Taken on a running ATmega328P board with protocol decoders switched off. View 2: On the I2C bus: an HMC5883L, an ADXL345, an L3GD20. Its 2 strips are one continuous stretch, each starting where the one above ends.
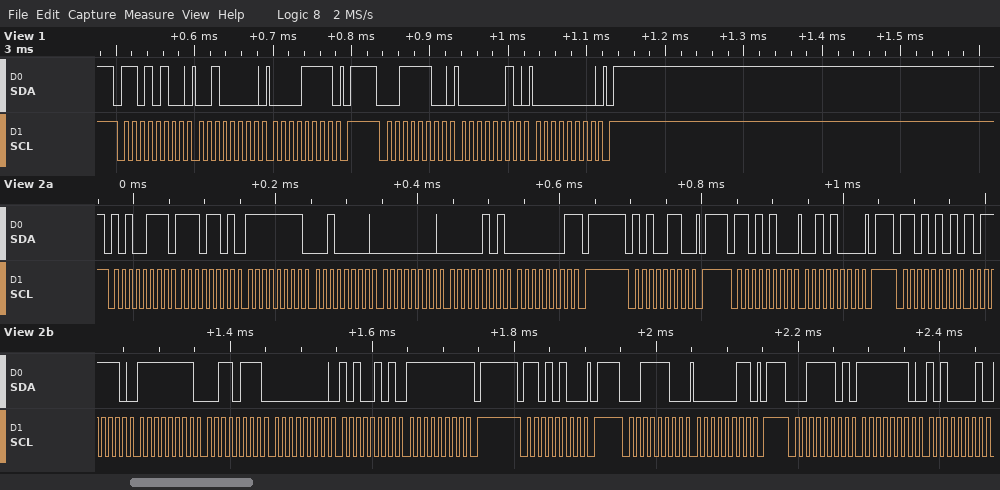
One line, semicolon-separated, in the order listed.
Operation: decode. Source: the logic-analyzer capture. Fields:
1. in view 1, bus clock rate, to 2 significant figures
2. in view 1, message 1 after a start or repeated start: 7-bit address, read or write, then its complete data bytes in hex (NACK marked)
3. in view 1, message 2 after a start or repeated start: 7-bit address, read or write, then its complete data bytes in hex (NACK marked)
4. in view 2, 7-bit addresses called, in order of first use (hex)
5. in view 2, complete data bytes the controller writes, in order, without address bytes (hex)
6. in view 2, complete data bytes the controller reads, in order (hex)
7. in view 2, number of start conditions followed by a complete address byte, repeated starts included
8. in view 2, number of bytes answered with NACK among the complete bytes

100 kHz; 0x6A write: 20 0F; 0x1E write: 02 00; 0x53 0x6A 0x1E; 28 03; ED FF 20 00 05 01 BE FF 37 00 A5 FF FE A1; 7; 2
